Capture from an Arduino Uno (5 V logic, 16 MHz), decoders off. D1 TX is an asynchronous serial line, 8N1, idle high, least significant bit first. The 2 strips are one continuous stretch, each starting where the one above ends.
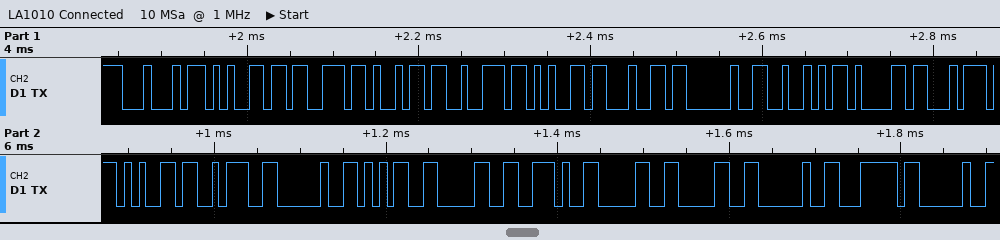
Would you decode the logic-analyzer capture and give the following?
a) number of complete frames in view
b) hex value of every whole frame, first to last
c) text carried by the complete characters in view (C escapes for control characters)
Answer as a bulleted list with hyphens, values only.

- 22
- 44 65 73 69 72 65 64 20 52 61 74 65 3A 20 35 30 2E 30 30 20 7C 20
- "Desired Rate: 50.00 | "
